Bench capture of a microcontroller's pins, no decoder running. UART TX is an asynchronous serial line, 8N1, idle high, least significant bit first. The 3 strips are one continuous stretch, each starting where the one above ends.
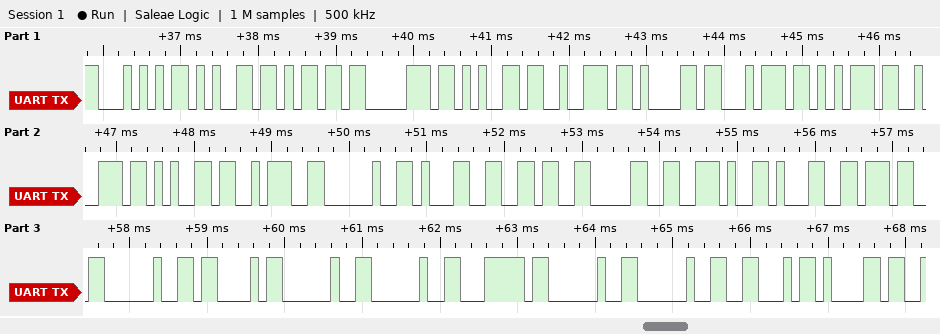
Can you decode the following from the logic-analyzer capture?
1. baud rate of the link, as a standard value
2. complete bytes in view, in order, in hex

9600 baud
54 65 6D 70 65 72 61 74 75 72 65 3A 20 31 36 30 2E 31 37 20 43 20 20 7C 20 20 46 61
